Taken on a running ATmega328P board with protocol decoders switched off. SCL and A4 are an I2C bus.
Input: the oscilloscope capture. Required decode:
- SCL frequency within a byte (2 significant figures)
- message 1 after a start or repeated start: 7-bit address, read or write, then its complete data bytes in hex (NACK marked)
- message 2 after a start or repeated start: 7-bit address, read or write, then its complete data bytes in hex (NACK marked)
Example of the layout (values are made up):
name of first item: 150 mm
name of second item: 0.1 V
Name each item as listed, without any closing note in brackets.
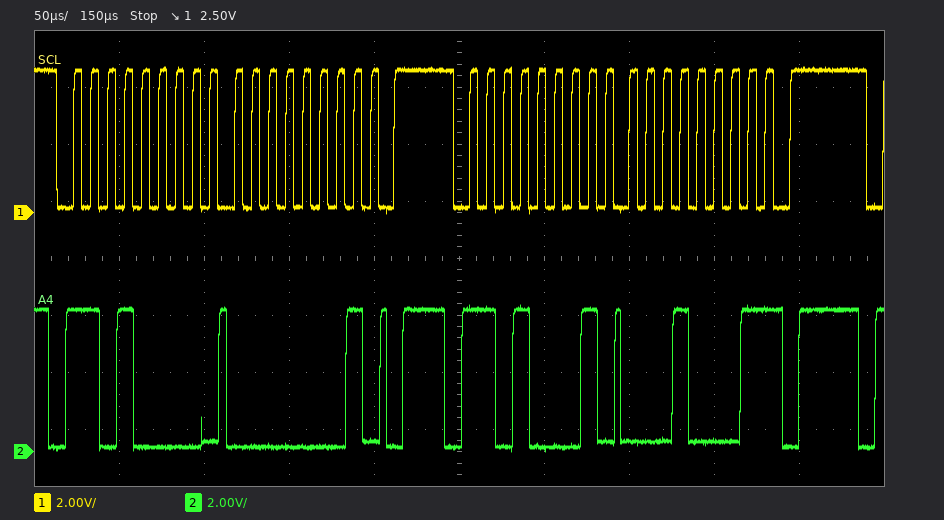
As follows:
SCL frequency within a byte: 100 kHz
message 1 after a start or repeated start: 7-bit address, read or write, then its complete data bytes in hex: 0x68 write: 01
message 2 after a start or repeated start: 7-bit address, read or write, then its complete data bytes in hex: 0x68 read: 11 NACK
